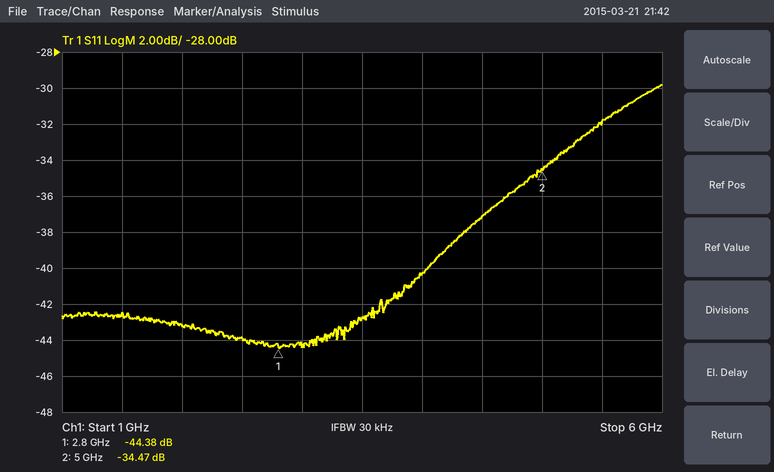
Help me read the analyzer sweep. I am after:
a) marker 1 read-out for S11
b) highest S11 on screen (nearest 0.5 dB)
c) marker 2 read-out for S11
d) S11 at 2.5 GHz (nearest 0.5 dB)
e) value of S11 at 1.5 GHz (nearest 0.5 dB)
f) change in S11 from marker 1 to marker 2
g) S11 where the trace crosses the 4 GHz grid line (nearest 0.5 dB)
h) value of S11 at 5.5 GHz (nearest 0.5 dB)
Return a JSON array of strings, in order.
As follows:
["-44.38 dB", "-30.0 dB", "-34.47 dB", "-44.0 dB", "-42.5 dB", "9.91 dB", "-40.5 dB", "-32.0 dB"]
